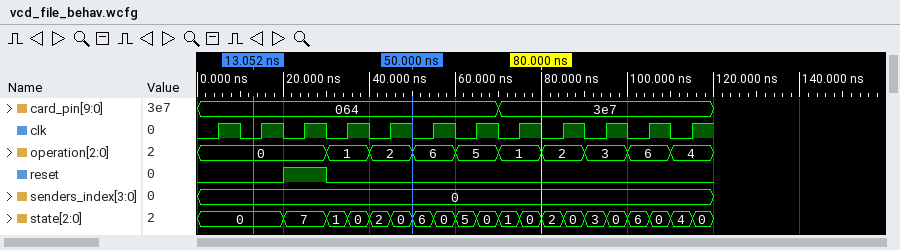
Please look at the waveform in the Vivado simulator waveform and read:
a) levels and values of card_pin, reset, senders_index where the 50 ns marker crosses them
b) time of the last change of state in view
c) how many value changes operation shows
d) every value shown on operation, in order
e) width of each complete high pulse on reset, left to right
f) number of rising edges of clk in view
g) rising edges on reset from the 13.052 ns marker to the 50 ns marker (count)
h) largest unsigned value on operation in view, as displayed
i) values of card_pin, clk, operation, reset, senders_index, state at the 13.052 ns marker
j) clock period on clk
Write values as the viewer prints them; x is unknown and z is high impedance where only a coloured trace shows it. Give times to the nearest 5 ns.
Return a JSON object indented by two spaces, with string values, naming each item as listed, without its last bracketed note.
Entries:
{
  "levels and values of card_pin, reset, senders_index where the 50 ns marker crosses them": "card_pin=064, reset=0, senders_index=0",
  "time of the last change of state in view": "115 ns",
  "how many value changes operation shows": "9",
  "every value shown on operation, in order": "0, 1, 2, 6, 5, 1, 2, 3, 6, 4",
  "width of each complete high pulse on reset, left to right": "10 ns",
  "number of rising edges of clk in view": "12",
  "rising edges on reset from the 13.052 ns marker to the 50 ns marker": "1",
  "largest unsigned value on operation in view, as displayed": "6",
  "values of card_pin, clk, operation, reset, senders_index, state at the 13.052 ns marker": "card_pin=064, clk=0, operation=0, reset=0, senders_index=0, state=0",
  "clock period on clk": "10 ns"
}
